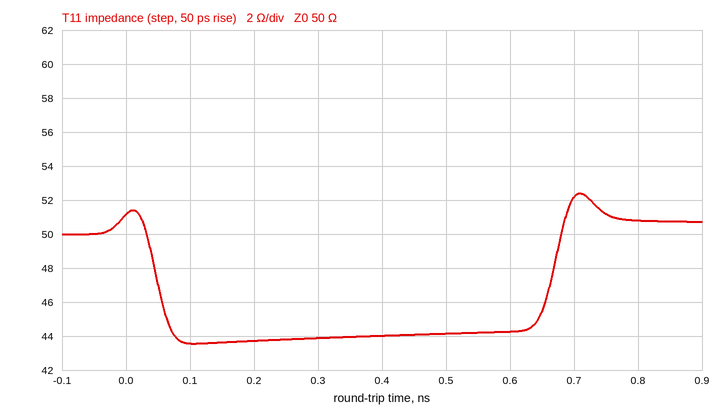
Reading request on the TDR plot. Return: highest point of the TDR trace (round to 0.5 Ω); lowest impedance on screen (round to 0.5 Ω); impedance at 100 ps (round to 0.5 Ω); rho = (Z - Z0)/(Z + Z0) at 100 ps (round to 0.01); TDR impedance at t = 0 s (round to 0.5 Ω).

52.5 Ω
43.5 Ω
43.5 Ω
-0.07
51.0 Ω
